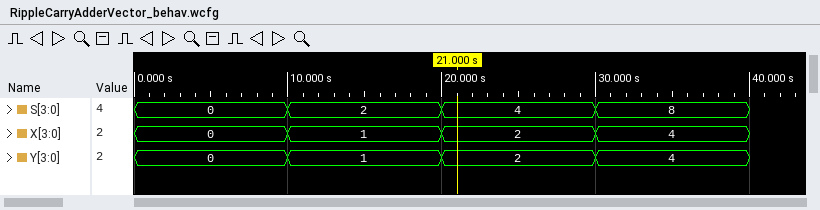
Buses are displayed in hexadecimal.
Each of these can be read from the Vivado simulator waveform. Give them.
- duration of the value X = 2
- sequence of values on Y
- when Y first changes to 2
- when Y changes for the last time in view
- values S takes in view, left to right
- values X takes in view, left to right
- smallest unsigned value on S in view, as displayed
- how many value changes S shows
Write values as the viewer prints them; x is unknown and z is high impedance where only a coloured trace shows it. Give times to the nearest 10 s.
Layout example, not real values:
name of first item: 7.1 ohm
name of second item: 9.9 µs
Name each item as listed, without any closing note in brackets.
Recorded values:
duration of the value X = 2: 10 s
sequence of values on Y: 0, 1, 2, 4
when Y first changes to 2: 20 s
when Y changes for the last time in view: 30 s
values S takes in view, left to right: 0, 2, 4, 8
values X takes in view, left to right: 0, 1, 2, 4
smallest unsigned value on S in view, as displayed: 0
how many value changes S shows: 3
